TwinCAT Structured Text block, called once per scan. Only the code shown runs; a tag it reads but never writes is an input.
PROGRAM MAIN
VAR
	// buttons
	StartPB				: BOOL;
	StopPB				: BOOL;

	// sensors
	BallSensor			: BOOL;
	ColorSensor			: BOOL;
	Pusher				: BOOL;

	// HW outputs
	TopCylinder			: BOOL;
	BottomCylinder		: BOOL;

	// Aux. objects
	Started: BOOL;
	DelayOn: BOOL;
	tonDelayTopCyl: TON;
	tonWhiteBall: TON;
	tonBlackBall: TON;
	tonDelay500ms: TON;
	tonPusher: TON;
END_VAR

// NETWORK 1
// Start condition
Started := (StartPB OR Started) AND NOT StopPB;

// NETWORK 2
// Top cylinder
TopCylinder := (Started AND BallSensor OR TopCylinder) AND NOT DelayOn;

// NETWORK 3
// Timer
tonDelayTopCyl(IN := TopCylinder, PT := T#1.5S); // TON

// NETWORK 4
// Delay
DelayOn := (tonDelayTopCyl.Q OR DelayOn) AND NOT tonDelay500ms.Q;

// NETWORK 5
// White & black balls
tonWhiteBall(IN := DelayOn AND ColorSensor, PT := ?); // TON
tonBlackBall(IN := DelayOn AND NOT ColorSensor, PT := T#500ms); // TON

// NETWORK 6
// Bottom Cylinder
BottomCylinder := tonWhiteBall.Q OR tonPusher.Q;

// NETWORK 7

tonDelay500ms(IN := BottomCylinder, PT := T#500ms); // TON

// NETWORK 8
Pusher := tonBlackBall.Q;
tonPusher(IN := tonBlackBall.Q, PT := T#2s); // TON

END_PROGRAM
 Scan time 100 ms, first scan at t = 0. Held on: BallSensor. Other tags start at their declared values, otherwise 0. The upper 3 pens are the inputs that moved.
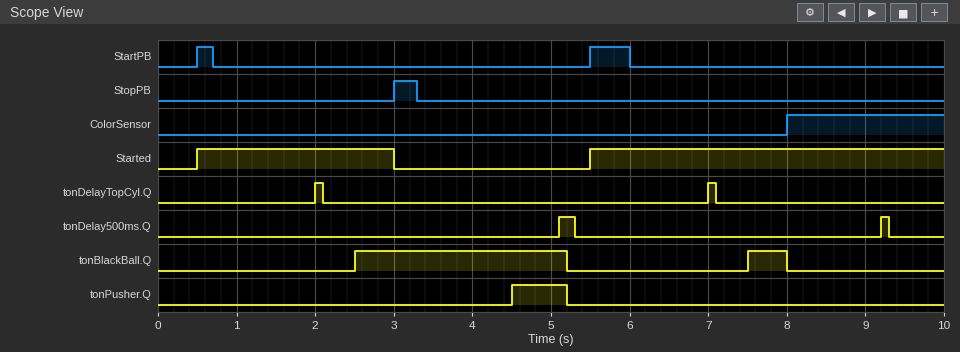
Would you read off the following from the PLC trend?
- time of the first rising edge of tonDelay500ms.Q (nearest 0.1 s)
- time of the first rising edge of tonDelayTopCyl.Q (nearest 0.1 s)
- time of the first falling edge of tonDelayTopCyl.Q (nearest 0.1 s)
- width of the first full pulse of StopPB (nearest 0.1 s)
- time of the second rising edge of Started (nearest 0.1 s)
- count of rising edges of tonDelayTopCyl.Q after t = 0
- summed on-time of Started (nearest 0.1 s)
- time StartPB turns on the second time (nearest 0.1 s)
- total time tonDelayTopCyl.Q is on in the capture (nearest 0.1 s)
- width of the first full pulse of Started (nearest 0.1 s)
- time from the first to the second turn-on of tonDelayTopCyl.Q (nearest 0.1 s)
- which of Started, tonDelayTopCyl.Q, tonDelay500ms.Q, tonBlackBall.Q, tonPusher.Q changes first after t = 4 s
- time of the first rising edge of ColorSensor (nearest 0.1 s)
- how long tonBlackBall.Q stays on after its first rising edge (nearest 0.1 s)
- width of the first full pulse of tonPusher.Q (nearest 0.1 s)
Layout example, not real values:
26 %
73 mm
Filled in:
5.1 s
2.0 s
2.1 s
0.3 s
5.5 s
2
7.0 s
5.5 s
0.2 s
2.5 s
5.0 s
tonPusher.Q
8.0 s
2.7 s
0.7 s
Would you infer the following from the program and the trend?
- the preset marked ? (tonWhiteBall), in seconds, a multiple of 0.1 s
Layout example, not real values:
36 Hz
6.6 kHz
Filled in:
0.7 s
